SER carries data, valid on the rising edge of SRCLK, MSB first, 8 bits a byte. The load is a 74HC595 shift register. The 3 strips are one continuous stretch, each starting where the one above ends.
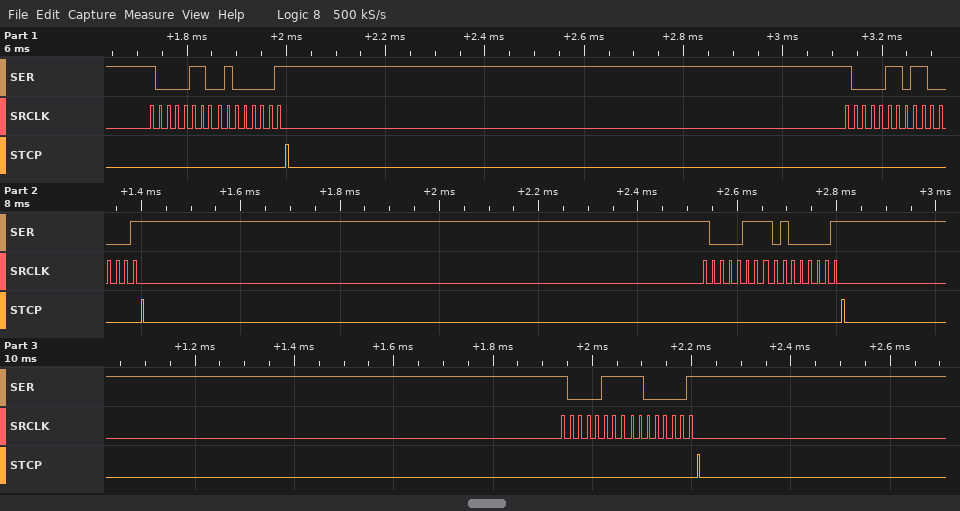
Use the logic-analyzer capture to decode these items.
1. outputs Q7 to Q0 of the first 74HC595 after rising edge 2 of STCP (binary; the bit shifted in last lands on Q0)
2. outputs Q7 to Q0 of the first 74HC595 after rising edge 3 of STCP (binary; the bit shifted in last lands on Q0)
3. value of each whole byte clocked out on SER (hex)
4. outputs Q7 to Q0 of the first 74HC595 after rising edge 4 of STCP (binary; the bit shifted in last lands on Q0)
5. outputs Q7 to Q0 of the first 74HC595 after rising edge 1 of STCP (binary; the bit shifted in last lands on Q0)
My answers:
11000001
01000001
86 41 86 C1 87 41 87 C1
11000001
01000001
